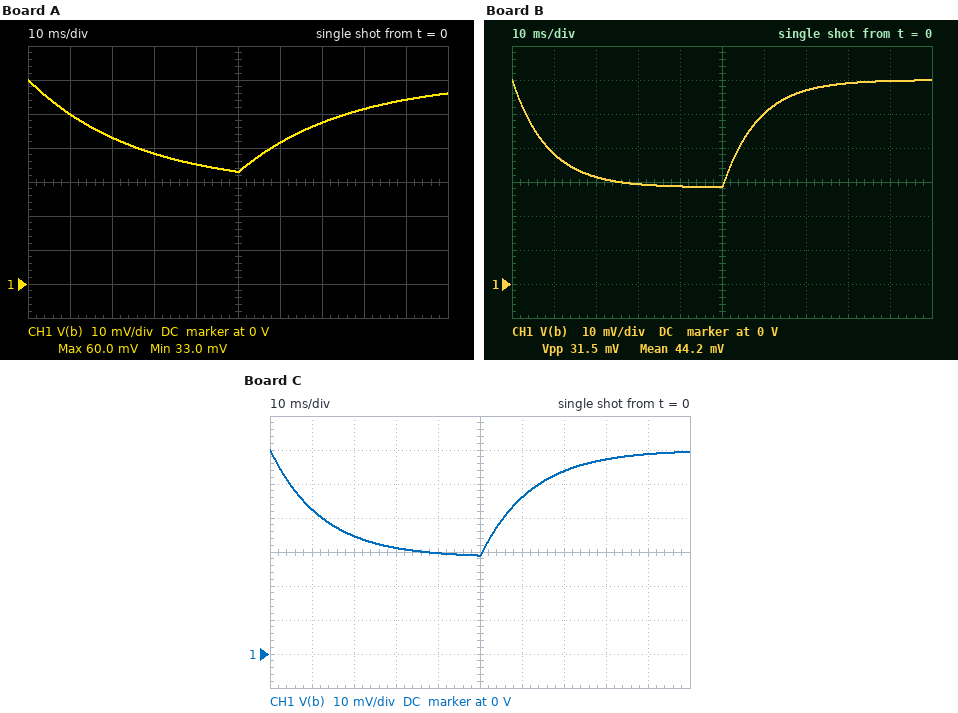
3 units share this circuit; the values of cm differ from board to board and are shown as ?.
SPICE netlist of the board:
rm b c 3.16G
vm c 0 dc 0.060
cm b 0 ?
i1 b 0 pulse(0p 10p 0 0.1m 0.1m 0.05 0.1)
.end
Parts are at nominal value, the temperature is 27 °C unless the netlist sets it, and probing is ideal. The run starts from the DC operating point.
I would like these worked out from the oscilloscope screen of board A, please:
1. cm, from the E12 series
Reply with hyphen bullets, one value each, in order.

- 8.2 pF
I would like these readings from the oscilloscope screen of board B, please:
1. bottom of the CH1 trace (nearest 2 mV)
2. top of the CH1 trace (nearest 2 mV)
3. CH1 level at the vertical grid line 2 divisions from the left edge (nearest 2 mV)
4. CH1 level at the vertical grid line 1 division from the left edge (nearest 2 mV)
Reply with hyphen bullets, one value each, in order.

- 28 mV
- 60 mV
- 32 mV
- 38 mV
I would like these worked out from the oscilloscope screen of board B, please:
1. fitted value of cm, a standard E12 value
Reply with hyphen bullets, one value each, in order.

- 2.7 pF
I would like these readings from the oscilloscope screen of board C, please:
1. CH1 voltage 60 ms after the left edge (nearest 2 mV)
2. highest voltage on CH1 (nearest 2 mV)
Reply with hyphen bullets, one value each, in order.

- 46 mV
- 60 mV
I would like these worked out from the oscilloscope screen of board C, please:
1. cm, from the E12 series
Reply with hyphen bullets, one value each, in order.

- 3.9 pF
